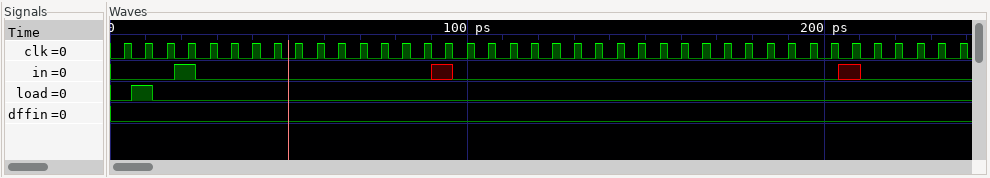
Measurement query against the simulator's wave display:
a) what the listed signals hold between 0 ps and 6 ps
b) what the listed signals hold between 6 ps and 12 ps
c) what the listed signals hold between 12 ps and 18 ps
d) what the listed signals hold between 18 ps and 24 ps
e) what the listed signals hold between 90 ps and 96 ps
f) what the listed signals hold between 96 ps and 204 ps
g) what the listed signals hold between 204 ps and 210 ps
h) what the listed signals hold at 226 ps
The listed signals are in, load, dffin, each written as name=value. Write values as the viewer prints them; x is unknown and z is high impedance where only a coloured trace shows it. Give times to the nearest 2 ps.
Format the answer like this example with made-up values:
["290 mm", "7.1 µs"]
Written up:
["in=0, load=0, dffin=0", "in=0, load=1, dffin=0", "in=0, load=0, dffin=0", "in=1, load=0, dffin=0", "in=x, load=0, dffin=0", "in=0, load=0, dffin=0", "in=x, load=0, dffin=0", "in=0, load=0, dffin=0"]
